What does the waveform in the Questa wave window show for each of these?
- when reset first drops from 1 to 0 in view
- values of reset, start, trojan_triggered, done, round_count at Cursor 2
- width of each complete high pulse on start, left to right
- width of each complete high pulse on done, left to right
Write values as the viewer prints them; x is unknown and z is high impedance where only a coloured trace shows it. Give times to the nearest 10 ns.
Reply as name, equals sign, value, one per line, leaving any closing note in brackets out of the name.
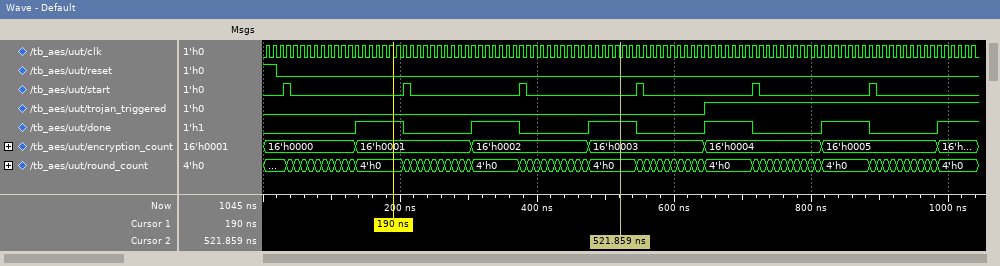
when reset first drops from 1 to 0 in view = 20 ns
values of reset, start, trojan_triggered, done, round_count at Cursor 2 = reset=0, start=0, trojan_triggered=0, done=1, round_count=4'h0
width of each complete high pulse on start, left to right = 10 ns, 10 ns, 10 ns, 10 ns, 10 ns, 10 ns
width of each complete high pulse on done, left to right = 70 ns, 70 ns, 70 ns, 70 ns, 70 ns
